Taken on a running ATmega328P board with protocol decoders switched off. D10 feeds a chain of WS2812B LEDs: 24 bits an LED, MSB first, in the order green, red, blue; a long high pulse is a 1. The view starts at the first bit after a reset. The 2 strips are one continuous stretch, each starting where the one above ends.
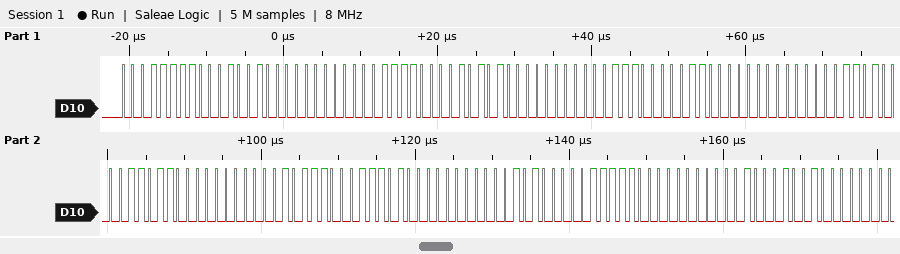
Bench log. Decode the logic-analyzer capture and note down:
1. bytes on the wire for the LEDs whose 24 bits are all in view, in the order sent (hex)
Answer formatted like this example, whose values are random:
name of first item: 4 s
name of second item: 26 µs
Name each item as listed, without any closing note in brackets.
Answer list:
bytes on the wire for the LEDs whose 24 bits are all in view, in the order sent: 1F 12 00 1E 15 00 1C 18 00 1A 1B 00 17 1D 00 14 1F 00
